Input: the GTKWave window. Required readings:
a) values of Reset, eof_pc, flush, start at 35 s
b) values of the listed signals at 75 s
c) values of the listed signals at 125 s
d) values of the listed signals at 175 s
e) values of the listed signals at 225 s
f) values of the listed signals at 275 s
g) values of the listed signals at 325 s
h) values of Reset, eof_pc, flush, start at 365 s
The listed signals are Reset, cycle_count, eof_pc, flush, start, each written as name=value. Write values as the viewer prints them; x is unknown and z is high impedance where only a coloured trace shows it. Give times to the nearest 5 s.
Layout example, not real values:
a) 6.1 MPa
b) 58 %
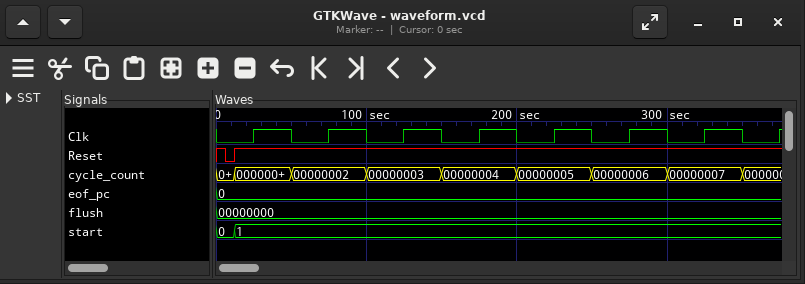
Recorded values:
a) Reset=1, eof_pc=0, flush=00000000, start=1
b) Reset=1, cycle_count=00000002, eof_pc=0, flush=00000000, start=1
c) Reset=1, cycle_count=00000003, eof_pc=0, flush=00000000, start=1
d) Reset=1, cycle_count=00000004, eof_pc=0, flush=00000000, start=1
e) Reset=1, cycle_count=00000005, eof_pc=0, flush=00000000, start=1
f) Reset=1, cycle_count=00000006, eof_pc=0, flush=00000000, start=1
g) Reset=1, cycle_count=00000007, eof_pc=0, flush=00000000, start=1
h) Reset=1, eof_pc=0, flush=00000000, start=1
